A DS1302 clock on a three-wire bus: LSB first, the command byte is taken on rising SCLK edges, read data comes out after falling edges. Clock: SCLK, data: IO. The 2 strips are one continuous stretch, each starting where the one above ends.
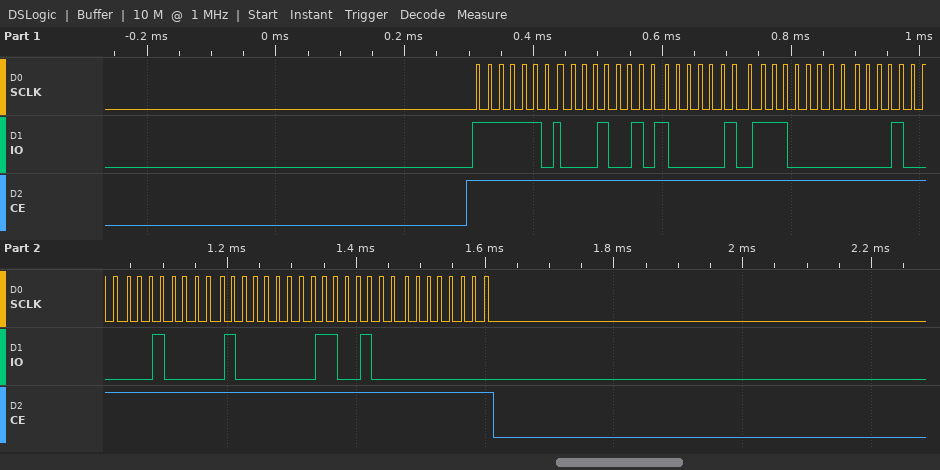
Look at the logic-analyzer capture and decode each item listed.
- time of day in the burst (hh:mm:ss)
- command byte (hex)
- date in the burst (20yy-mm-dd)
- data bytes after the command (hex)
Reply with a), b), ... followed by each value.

a) 07:41:48
b) 0xBF
c) 2026-08-10
d) 48 41 07 10 08 02 26 00
